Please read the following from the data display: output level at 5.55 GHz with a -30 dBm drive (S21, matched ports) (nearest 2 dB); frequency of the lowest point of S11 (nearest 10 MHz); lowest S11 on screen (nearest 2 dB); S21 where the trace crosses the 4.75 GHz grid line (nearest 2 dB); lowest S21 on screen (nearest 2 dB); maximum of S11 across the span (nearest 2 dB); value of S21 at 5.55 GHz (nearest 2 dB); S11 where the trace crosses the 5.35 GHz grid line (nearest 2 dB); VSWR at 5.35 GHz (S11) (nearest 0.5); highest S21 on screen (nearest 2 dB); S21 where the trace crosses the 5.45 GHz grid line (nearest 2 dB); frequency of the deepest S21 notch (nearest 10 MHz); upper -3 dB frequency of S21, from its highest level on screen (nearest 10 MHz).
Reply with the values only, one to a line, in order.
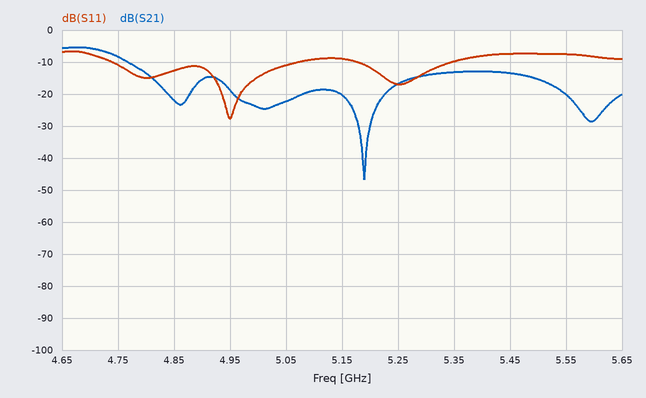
-50 dBm
4.95 GHz
-28 dB
-8 dB
-46 dB
-6 dB
-20 dB
-10 dB
2.0
-6 dB
-14 dB
5.19 GHz
4.75 GHz
